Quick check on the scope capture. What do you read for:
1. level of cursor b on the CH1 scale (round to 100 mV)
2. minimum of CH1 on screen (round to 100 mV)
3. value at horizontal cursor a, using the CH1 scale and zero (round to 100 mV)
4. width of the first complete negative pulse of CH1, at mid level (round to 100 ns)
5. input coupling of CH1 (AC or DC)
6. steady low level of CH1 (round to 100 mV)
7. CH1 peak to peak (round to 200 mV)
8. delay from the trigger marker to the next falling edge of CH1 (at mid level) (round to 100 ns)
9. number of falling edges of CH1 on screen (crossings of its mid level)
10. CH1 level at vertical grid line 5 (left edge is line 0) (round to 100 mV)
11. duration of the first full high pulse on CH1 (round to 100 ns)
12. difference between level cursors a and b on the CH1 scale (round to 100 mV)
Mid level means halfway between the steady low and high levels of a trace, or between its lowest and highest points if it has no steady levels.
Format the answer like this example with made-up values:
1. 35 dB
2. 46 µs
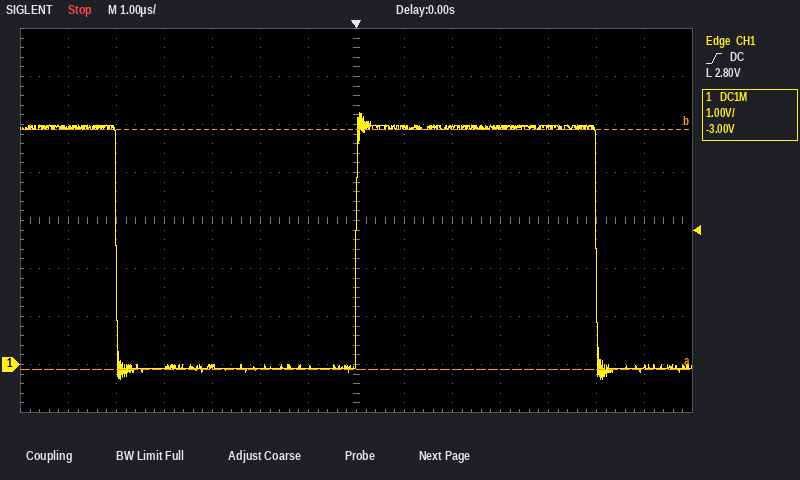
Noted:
1. 4.9 V
2. -300 mV
3. -100 mV
4. 5.0 µs
5. DC
6. -100 mV
7. 5.6 V
8. 5.0 µs
9. 2
10. -100 mV
11. 5.0 µs
12. 5.0 V
